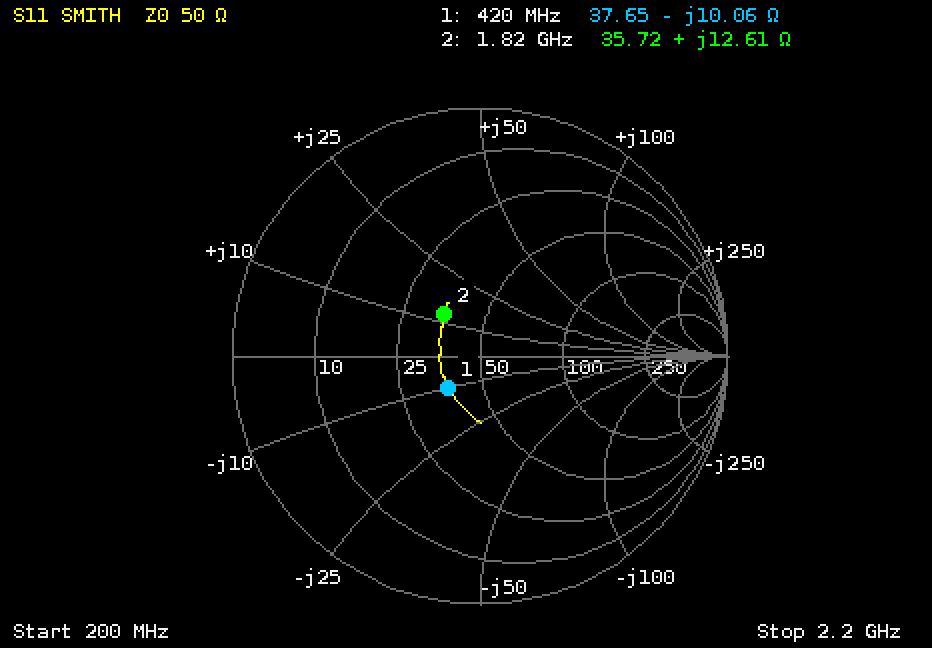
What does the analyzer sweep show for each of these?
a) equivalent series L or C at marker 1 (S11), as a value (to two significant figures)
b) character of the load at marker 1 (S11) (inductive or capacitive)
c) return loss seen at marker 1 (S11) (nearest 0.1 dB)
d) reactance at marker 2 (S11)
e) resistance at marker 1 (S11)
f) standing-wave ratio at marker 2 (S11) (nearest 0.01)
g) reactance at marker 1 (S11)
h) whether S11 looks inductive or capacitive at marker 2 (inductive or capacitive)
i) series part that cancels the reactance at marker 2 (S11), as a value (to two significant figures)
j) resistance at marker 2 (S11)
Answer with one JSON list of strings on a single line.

["38 pF", "capacitive", "14.9 dB", "+12.61 Ω", "37.65 Ω", "1.56", "-10.06 Ω", "inductive", "6.9 pF", "35.72 Ω"]
